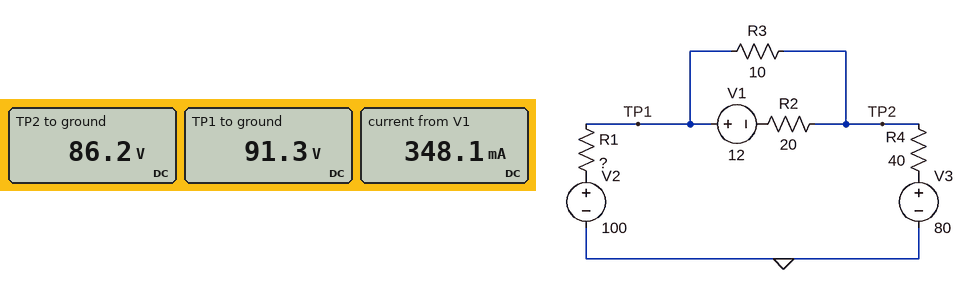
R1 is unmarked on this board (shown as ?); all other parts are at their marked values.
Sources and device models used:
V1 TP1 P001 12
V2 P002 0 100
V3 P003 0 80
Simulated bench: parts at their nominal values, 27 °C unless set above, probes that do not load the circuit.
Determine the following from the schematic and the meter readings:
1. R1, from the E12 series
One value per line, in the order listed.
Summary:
56 Ω
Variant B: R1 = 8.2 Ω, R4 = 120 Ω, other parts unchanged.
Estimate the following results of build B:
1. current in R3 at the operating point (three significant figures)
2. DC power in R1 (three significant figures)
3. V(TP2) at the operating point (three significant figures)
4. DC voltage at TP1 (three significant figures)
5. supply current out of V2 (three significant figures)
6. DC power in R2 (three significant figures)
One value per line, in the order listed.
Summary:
479 mA
115 mW
94.2 V
99.0 V
119 mA
2.60 W
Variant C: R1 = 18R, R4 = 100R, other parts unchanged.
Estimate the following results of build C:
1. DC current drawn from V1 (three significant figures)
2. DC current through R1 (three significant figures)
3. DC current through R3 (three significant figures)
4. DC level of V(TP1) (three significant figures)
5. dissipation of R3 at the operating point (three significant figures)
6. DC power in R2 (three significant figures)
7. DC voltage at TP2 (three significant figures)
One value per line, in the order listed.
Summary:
357 mA
128 mA
486 mA
97.7 V
2.36 W
2.55 W
92.8 V
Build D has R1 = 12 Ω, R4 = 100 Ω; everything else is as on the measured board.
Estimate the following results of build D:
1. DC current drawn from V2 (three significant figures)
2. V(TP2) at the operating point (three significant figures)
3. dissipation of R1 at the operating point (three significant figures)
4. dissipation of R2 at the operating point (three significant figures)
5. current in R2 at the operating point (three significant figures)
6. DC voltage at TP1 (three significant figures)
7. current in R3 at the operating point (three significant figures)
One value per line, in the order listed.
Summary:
135 mA
93.5 V
218 mW
2.52 W
355 mA
98.4 V
490 mA
